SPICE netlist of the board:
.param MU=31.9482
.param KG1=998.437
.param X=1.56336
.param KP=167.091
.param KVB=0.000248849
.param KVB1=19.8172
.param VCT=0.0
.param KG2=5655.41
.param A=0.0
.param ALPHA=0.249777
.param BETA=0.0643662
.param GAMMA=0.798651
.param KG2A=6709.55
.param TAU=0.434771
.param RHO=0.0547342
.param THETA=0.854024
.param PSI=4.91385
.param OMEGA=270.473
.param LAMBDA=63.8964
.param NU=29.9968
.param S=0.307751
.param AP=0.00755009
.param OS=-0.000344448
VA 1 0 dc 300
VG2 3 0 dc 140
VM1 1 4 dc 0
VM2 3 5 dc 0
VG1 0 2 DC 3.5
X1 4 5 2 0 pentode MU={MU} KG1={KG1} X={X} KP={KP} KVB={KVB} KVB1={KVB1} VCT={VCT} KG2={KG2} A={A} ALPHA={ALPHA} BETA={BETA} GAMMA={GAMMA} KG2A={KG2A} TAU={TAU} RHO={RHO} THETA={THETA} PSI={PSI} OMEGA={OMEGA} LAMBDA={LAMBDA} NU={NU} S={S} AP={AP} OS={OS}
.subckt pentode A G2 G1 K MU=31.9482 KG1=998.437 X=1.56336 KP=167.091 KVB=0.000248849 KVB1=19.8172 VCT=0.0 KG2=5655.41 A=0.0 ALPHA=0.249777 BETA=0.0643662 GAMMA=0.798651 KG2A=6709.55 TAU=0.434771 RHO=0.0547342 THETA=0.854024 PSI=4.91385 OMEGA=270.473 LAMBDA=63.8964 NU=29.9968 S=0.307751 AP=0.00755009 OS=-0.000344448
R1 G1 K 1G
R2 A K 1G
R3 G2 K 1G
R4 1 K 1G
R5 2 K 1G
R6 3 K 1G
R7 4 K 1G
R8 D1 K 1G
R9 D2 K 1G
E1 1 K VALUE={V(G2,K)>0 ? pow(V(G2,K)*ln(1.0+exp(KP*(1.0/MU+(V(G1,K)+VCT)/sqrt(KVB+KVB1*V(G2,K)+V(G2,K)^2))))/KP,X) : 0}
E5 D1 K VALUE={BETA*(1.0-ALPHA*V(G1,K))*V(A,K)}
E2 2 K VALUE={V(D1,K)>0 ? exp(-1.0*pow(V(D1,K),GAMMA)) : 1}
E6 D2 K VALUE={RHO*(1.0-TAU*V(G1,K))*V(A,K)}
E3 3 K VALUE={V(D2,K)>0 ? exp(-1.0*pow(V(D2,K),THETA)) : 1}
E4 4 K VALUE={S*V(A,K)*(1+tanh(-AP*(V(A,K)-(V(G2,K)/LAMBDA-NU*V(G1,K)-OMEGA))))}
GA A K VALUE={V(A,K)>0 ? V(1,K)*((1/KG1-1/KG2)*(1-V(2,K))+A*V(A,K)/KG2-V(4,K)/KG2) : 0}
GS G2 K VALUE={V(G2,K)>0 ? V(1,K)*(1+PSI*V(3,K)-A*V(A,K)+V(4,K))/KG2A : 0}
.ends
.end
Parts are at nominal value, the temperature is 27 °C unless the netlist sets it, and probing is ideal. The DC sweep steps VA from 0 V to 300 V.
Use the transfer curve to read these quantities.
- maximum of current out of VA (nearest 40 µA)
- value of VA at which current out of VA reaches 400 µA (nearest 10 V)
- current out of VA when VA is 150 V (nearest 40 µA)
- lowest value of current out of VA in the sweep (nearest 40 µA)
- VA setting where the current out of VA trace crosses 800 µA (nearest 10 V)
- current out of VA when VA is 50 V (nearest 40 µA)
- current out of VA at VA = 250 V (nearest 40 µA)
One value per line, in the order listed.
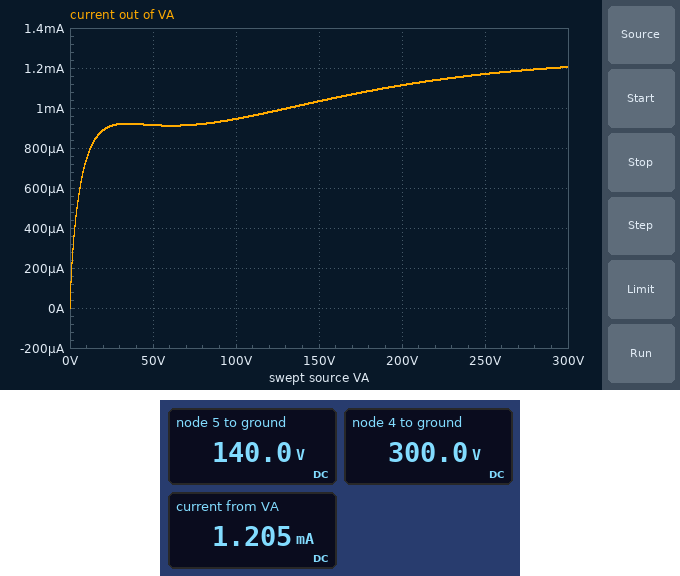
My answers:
1.20 mA
0 V
1.04 mA
0 A
10 V
920 µA
1.16 mA
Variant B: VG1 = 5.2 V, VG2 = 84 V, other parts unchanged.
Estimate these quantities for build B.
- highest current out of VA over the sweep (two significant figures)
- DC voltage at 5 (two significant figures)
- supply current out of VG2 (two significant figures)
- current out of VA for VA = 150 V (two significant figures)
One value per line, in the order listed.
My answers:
740 nA
84 V
200 nA
450 nA
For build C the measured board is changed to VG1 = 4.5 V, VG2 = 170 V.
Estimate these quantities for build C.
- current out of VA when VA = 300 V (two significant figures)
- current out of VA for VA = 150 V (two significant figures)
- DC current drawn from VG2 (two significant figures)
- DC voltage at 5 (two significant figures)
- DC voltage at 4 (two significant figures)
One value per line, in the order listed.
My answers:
1.3 mA
980 µA
310 µA
170 V
300 V
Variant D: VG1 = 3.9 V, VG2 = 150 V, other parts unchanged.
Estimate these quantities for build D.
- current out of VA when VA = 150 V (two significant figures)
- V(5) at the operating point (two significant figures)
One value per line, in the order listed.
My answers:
960 µA
150 V
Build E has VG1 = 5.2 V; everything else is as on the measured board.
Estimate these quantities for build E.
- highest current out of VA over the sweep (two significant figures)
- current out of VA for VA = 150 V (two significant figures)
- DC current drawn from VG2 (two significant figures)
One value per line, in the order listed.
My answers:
160 µA
110 µA
44 µA
